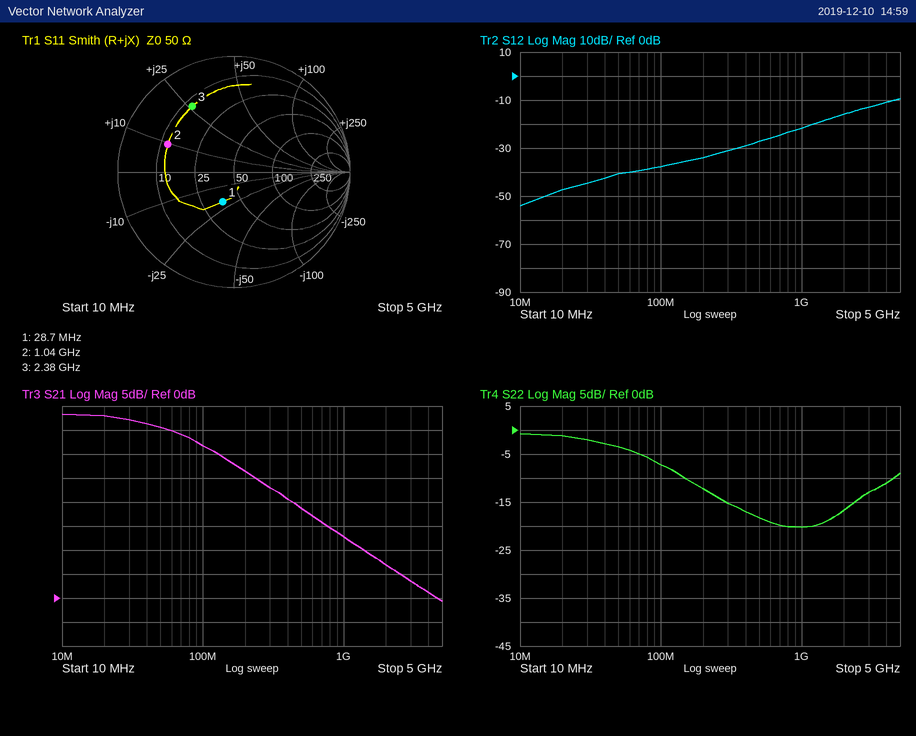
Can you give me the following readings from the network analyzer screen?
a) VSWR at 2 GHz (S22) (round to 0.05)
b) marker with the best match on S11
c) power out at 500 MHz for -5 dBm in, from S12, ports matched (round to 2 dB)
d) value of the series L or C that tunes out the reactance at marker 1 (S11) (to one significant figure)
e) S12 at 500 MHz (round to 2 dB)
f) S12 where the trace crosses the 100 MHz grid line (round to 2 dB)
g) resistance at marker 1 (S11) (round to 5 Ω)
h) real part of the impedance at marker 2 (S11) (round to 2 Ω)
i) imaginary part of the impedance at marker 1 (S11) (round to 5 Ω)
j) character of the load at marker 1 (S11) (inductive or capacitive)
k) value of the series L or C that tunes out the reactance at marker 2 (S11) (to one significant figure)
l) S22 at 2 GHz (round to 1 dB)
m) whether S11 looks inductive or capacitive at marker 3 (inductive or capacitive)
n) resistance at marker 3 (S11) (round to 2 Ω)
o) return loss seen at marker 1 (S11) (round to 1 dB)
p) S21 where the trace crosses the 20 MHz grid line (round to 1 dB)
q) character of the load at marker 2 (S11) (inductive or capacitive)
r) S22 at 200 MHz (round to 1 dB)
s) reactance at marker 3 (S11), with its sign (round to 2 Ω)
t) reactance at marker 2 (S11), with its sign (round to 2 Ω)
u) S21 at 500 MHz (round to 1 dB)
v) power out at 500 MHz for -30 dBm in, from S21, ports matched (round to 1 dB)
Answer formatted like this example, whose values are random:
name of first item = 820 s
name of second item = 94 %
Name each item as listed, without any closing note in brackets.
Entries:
VSWR at 2 GHz (S22) = 1.35
marker with the best match on S11 = marker 1
power out at 500 MHz for -5 dBm in, from S12, ports matched = -32 dBm
value of the series L or C that tunes out the reactance at marker 1 (S11) = 100 nH
S12 at 500 MHz = -28 dB
S12 where the trace crosses the 100 MHz grid line = -38 dB
resistance at marker 1 (S11) = 35 Ω
real part of the impedance at marker 2 (S11) = 12 Ω
imaginary part of the impedance at marker 1 (S11) = -20 Ω
character of the load at marker 1 (S11) = capacitive
value of the series L or C that tunes out the reactance at marker 2 (S11) = 20 pF
S22 at 2 GHz = -17 dB
whether S11 looks inductive or capacitive at marker 3 = inductive
resistance at marker 3 (S11) = 12 Ω
return loss seen at marker 1 (S11) = 11 dB
S21 where the trace crosses the 20 MHz grid line = 38 dB
character of the load at marker 2 (S11) = inductive
S22 at 200 MHz = -12 dB
reactance at marker 3 (S11), with its sign = +26 Ω
reactance at marker 2 (S11), with its sign = +10 Ω
S21 at 500 MHz = 19 dB
power out at 500 MHz for -30 dBm in, from S21, ports matched = -11 dBm
